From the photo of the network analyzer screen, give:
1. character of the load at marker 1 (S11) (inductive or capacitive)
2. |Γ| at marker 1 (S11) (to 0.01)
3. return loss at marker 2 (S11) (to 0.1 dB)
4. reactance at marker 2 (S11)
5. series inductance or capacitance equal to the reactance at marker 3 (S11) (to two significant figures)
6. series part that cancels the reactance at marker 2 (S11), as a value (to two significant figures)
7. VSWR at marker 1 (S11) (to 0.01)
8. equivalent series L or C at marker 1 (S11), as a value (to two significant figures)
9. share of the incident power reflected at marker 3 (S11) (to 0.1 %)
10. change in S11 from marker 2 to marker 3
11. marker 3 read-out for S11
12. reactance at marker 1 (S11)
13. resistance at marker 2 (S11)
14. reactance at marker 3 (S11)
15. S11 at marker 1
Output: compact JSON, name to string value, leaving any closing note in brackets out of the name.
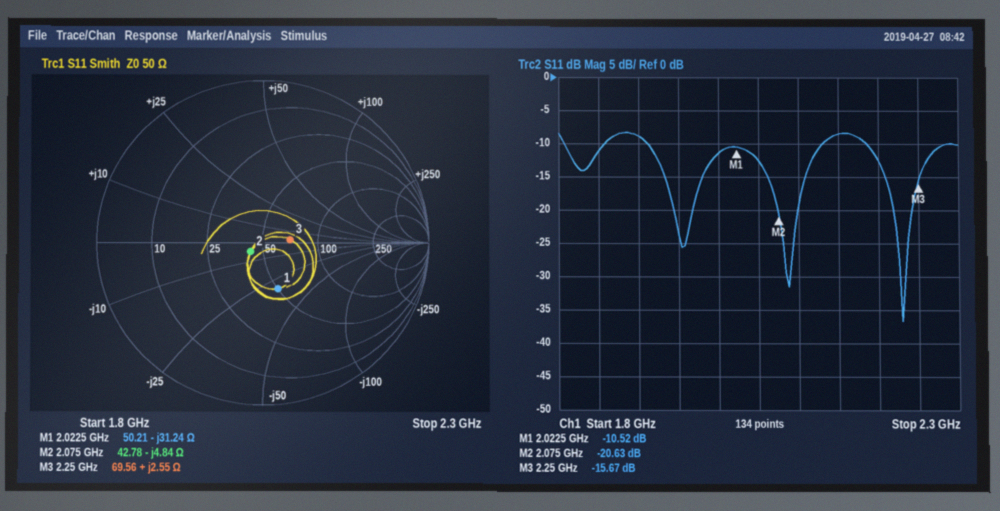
{"character of the load at marker 1 (S11)": "capacitive", "|Γ| at marker 1 (S11)": "0.30", "return loss at marker 2 (S11)": "20.6 dB", "reactance at marker 2": "-4.84 Ω", "series inductance or capacitance equal to the reactance at marker 3 (S11)": "180 pH", "series part that cancels the reactance at marker 2 (S11), as a value": "370 pH", "VSWR at marker 1 (S11)": "1.85", "equivalent series L or C at marker 1 (S11), as a value": "2.5 pF", "share of the incident power reflected at marker 3 (S11)": "2.7 %", "change in S11 from marker 2 to marker 3": "4.96 dB", "marker 3 read-out for S11": "-15.67 dB", "reactance at marker 1": "-31.24 Ω", "resistance at marker 2": "42.78 Ω", "reactance at marker 3": "+2.55 Ω", "S11 at marker 1": "-10.52 dB"}
